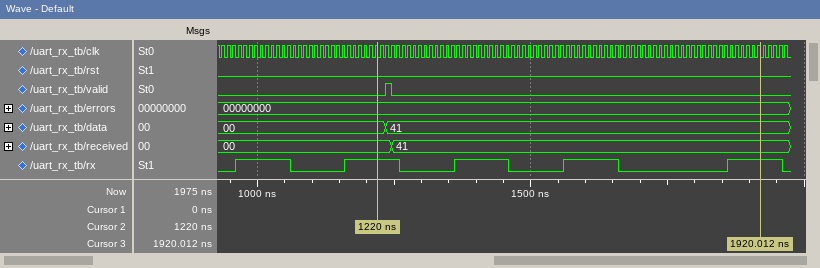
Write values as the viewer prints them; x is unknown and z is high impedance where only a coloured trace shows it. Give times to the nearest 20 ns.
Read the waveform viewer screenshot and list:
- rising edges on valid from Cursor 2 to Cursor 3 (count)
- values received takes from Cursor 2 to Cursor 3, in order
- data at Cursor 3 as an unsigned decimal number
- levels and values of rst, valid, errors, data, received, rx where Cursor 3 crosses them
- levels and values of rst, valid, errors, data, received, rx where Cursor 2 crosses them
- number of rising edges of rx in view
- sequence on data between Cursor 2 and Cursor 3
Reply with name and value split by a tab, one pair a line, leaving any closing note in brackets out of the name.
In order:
rising edges on valid from Cursor 2 to Cursor 3	1
values received takes from Cursor 2 to Cursor 3, in order	00, 41
data at Cursor 3 as an unsigned decimal number	65
levels and values of rst, valid, errors, data, received, rx where Cursor 3 crosses them	rst=0, valid=0, errors=00000000, data=41, received=41, rx=1
levels and values of rst, valid, errors, data, received, rx where Cursor 2 crosses them	rst=0, valid=0, errors=00000000, data=00, received=00, rx=1
number of rising edges of rx in view	5
sequence on data between Cursor 2 and Cursor 3	00, 41
